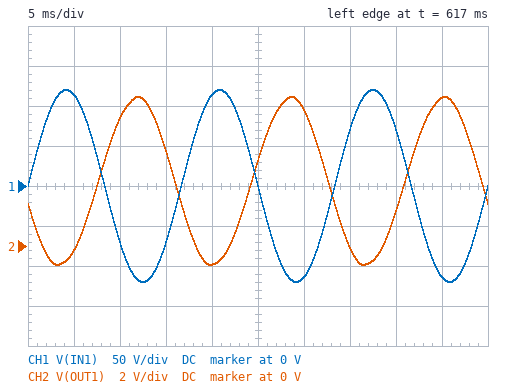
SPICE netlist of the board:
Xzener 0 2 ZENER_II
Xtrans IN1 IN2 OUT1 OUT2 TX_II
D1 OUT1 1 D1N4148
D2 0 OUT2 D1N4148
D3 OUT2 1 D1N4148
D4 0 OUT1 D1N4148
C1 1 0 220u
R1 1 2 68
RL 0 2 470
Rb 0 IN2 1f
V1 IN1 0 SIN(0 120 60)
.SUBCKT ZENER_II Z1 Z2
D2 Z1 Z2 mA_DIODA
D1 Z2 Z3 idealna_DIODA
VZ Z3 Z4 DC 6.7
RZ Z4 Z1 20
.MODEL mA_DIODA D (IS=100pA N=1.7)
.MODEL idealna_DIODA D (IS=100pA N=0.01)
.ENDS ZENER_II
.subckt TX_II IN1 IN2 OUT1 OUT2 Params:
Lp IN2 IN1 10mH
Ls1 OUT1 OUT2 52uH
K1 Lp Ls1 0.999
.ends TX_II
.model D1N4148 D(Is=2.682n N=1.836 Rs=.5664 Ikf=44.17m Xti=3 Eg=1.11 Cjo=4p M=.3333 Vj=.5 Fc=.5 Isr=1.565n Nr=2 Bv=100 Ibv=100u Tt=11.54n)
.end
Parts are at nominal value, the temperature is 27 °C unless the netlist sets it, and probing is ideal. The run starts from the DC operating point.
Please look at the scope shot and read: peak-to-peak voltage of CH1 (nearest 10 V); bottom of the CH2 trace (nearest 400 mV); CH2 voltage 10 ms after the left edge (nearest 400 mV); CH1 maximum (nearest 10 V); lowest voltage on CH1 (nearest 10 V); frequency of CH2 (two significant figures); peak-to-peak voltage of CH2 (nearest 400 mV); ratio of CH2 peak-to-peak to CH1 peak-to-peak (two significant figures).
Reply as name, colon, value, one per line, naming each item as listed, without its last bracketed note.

peak-to-peak voltage of CH1: 240 V
bottom of the CH2 trace: -800 mV
CH2 voltage 10 ms after the left edge: 6.4 V
CH1 maximum: 120 V
lowest voltage on CH1: -120 V
frequency of CH2: 60 Hz
peak-to-peak voltage of CH2: 8.4 V
ratio of CH2 peak-to-peak to CH1 peak-to-peak: 0.035
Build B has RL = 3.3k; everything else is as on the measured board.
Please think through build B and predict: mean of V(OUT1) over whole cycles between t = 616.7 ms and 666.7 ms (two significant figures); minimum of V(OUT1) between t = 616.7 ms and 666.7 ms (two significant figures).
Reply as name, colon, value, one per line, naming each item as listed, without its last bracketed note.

mean of V(OUT1) over whole cycles between t = 616.7 ms and 666.7 ms: 3.4 V
minimum of V(OUT1) between t = 616.7 ms and 666.7 ms: -790 mV
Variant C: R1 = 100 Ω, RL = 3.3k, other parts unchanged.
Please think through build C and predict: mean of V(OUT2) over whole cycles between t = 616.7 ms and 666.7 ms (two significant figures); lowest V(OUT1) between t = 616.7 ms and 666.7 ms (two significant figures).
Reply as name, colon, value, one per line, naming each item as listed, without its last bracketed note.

mean of V(OUT2) over whole cycles between t = 616.7 ms and 666.7 ms: 3.4 V
lowest V(OUT1) between t = 616.7 ms and 666.7 ms: -790 mV
